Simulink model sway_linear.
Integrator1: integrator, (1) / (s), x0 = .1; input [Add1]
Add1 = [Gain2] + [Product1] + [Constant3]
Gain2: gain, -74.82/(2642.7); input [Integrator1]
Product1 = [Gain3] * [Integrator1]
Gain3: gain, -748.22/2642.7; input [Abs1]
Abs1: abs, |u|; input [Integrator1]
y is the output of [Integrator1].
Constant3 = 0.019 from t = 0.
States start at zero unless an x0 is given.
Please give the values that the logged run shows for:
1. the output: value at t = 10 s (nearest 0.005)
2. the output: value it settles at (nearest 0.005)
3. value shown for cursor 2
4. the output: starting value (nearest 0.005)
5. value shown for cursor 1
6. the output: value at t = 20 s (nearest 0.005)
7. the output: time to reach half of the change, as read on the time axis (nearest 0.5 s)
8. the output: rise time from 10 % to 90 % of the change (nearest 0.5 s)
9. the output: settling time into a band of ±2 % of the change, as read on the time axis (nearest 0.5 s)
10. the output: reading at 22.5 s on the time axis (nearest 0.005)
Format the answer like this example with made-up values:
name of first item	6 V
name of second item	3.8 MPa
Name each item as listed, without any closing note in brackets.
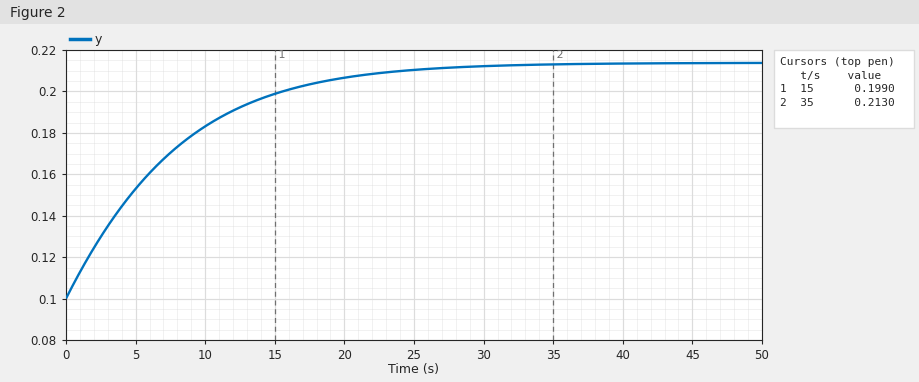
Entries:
the output: value at t = 10 s	0.185
the output: value it settles at	0.215
value shown for cursor 2	0.2130
the output: starting value	0.100
value shown for cursor 1	0.1990
the output: value at t = 20 s	0.205
the output: time to reach half of the change, as read on the time axis	5.5 s
the output: rise time from 10 % to 90 % of the change	16.0 s
the output: settling time into a band of ±2 % of the change, as read on the time axis	28.0 s
the output: reading at 22.5 s on the time axis	0.210
